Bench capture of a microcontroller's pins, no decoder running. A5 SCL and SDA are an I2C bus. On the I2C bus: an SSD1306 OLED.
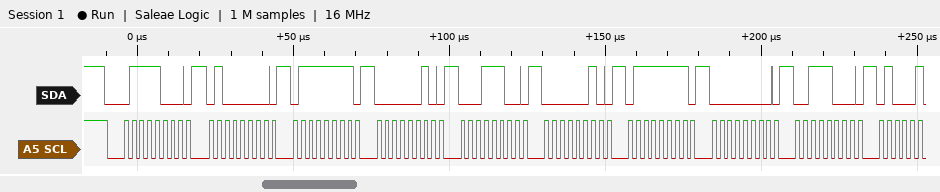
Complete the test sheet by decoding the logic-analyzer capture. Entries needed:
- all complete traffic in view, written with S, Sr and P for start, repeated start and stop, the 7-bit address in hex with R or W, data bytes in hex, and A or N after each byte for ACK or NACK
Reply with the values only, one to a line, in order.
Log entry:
S 3CW A 40 A 7F A 02 A 1C A 02 A 7F A 00 A 38 A
